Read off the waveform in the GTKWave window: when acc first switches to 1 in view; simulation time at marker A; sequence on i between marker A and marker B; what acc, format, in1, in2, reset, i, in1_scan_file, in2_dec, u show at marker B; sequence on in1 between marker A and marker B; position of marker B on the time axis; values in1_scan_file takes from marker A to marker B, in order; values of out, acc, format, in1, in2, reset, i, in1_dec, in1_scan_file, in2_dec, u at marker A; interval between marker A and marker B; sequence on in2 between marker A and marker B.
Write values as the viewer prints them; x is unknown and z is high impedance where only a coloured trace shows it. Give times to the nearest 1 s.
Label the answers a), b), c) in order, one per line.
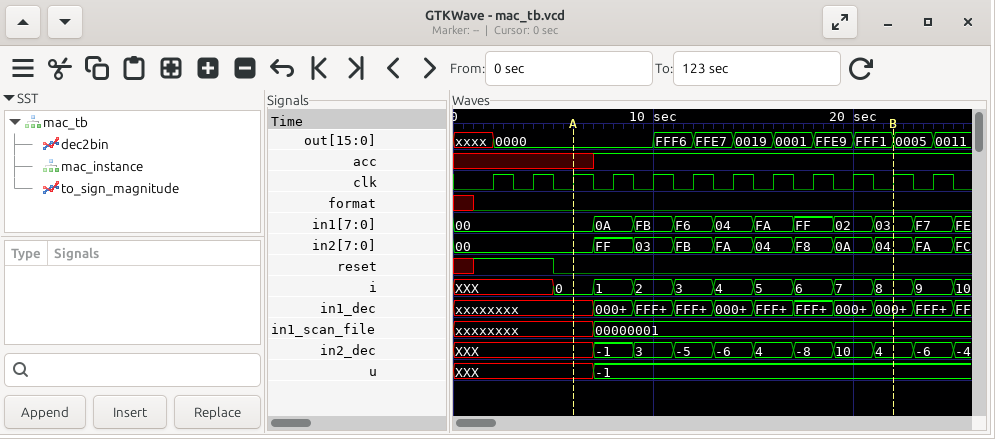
a) 7 s
b) 6 s
c) 0, 1, 2, 3, 4, 5, 6, 7, 8
d) acc=1, format=0, in1=03, in2=04, reset=0, i=8, in1_scan_file=00000001, in2_dec=4, u=-1
e) 00, 0A, FB, F6, 04, FA, FF, 02, 03
f) 22 s
g) xxxxxxxx, 00000001
h) out=0000, acc=x, format=0, in1=00, in2=00, reset=0, i=0, in1_dec=xxxxxxxx, in1_scan_file=xxxxxxxx, in2_dec=XXX, u=XXX
i) 16 s
j) 00, FF, 03, FB, FA, 04, F8, 0A, 04
